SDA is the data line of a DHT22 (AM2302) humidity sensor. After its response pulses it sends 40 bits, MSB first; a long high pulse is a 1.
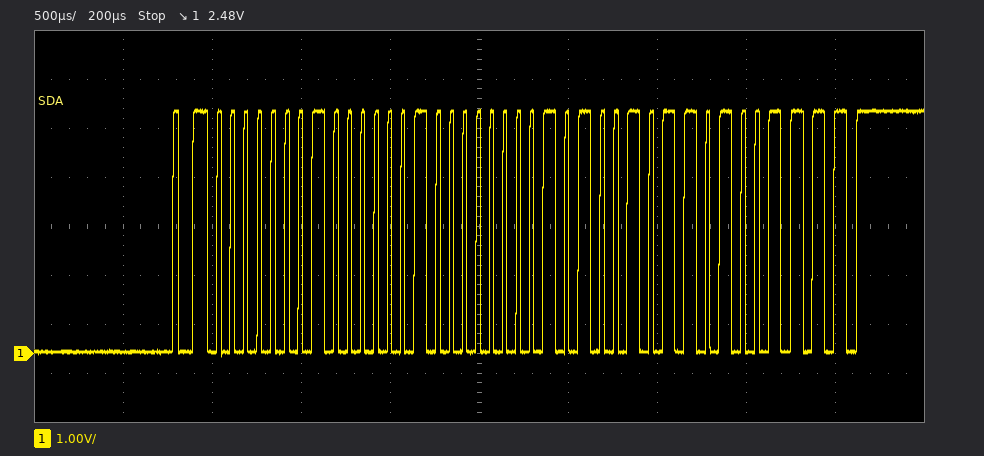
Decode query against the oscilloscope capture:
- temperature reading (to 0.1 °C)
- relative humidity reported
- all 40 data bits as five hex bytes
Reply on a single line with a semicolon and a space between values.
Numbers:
33.1 °C; 25.8 %; 01 02 01 4B 4F
